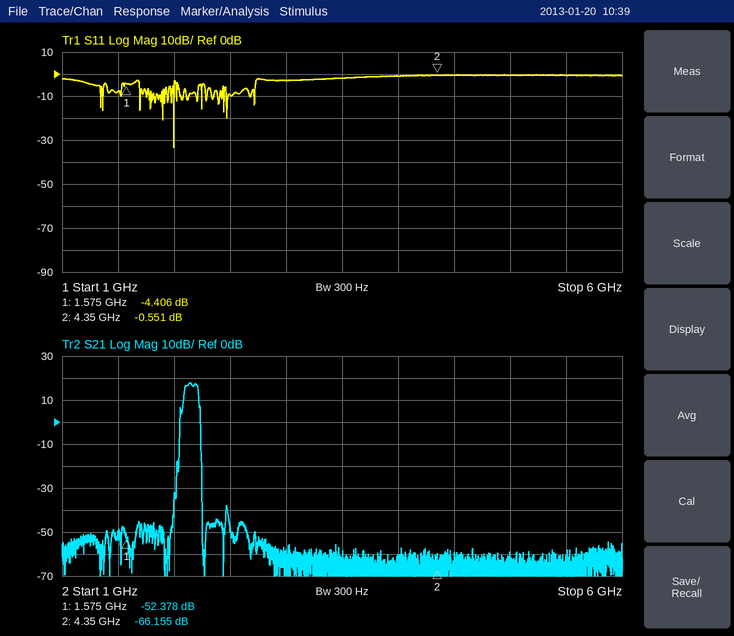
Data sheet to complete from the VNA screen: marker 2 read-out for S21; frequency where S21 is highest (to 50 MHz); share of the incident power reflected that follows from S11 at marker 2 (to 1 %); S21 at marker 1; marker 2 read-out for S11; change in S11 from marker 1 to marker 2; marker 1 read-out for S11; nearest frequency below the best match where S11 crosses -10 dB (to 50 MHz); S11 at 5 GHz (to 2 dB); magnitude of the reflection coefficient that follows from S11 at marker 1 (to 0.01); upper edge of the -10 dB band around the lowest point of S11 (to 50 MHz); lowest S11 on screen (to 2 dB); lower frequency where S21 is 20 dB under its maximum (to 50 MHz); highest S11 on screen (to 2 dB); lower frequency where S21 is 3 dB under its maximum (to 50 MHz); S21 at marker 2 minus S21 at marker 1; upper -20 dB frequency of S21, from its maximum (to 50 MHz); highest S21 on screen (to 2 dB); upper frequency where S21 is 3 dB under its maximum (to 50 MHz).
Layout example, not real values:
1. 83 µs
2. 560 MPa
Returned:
1. -66.155 dB
2. 2.15 GHz
3. 88 %
4. -52.378 dB
5. -0.551 dB
6. 3.855 dB
7. -4.406 dB
8. 2.00 GHz
9. 0 dB
10. 0.60
11. 2.00 GHz
12. -34 dB
13. 2.05 GHz
14. 0 dB
15. 2.10 GHz
16. -13.777 dB
17. 2.25 GHz
18. 18 dB
19. 2.20 GHz
